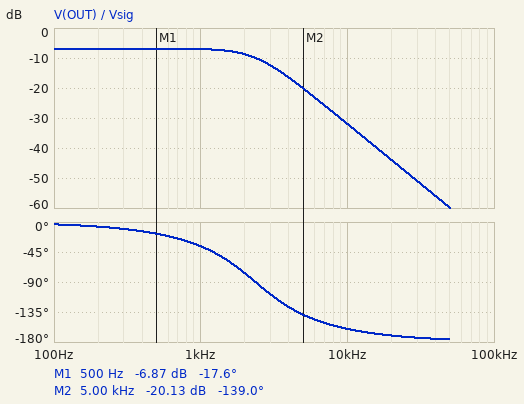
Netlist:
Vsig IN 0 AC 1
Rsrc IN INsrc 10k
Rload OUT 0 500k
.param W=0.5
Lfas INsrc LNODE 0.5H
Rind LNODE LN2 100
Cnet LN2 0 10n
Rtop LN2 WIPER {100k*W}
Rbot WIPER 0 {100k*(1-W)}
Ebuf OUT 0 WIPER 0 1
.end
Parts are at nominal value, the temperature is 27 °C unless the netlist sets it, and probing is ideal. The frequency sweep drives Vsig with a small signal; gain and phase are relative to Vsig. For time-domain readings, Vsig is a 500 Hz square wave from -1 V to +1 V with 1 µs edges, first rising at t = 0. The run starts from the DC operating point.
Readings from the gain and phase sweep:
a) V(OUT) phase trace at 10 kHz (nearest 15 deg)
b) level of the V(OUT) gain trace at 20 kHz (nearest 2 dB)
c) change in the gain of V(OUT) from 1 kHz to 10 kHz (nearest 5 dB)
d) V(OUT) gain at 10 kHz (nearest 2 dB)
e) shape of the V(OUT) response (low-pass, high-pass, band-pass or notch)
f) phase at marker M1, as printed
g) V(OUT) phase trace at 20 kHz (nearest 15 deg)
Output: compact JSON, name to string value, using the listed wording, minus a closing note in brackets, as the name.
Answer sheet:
{"V(OUT) phase trace at 10 kHz": "-165 deg", "level of the V(OUT) gain trace at 20 kHz": "-44 dB", "change in the gain of V(OUT) from 1 kHz to 10 kHz": "-25 dB", "V(OUT) gain at 10 kHz": "-32 dB", "shape of the V(OUT) response": "low-pass", "phase at marker M1, as printed": "-17.6 deg", "V(OUT) phase trace at 20 kHz": "-165 deg"}
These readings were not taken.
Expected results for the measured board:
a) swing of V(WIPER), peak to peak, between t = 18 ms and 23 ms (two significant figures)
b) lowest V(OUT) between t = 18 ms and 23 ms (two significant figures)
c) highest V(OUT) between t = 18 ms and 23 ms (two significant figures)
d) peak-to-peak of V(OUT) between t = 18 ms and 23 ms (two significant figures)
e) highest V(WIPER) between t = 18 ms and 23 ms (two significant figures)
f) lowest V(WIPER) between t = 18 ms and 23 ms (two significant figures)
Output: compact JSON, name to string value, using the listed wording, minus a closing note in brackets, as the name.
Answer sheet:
{"swing of V(WIPER), peak to peak, between t = 18 ms and 23 ms": "980 mV", "lowest V(OUT) between t = 18 ms and 23 ms": "-490 mV", "highest V(OUT) between t = 18 ms and 23 ms": "490 mV", "peak-to-peak of V(OUT) between t = 18 ms and 23 ms": "980 mV", "highest V(WIPER) between t = 18 ms and 23 ms": "490 mV", "lowest V(WIPER) between t = 18 ms and 23 ms": "-490 mV"}
